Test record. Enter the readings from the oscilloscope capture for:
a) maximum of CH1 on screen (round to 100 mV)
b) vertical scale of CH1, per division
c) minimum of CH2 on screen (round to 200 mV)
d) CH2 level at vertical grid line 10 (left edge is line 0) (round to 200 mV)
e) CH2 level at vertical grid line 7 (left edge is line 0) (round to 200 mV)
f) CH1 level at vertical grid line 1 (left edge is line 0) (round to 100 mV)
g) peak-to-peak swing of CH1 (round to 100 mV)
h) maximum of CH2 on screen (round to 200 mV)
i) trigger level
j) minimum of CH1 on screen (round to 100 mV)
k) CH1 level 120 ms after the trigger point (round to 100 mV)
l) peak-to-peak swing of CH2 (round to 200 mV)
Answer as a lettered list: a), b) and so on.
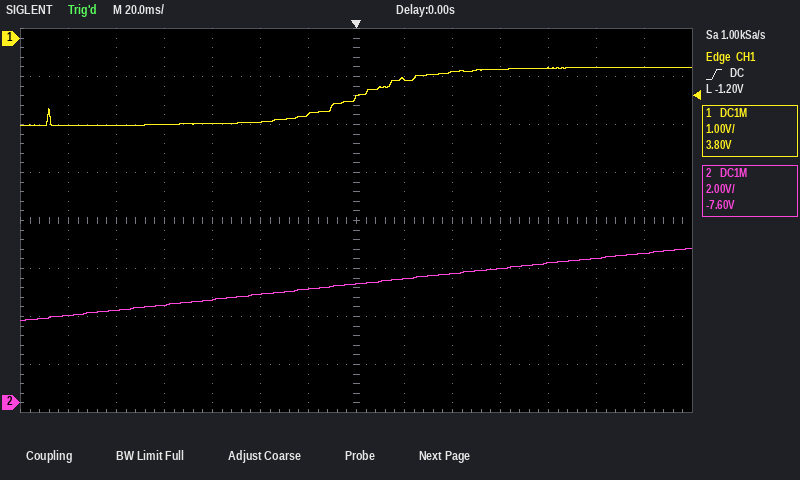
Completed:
a) -600 mV
b) 1 V
c) 3.4 V
d) 5.6 V
e) 5.0 V
f) -1.8 V
g) 1.2 V
h) 6.4 V
i) -1.20 V
j) -1.8 V
k) -600 mV
l) 3.0 V
